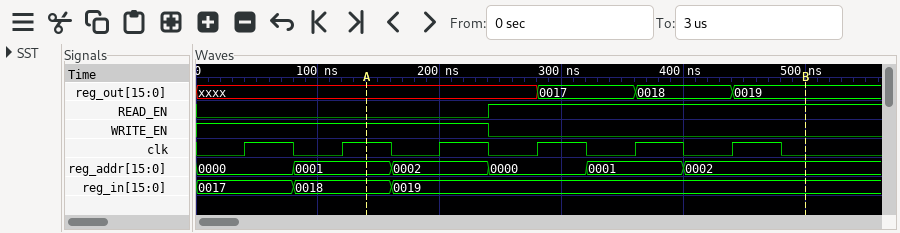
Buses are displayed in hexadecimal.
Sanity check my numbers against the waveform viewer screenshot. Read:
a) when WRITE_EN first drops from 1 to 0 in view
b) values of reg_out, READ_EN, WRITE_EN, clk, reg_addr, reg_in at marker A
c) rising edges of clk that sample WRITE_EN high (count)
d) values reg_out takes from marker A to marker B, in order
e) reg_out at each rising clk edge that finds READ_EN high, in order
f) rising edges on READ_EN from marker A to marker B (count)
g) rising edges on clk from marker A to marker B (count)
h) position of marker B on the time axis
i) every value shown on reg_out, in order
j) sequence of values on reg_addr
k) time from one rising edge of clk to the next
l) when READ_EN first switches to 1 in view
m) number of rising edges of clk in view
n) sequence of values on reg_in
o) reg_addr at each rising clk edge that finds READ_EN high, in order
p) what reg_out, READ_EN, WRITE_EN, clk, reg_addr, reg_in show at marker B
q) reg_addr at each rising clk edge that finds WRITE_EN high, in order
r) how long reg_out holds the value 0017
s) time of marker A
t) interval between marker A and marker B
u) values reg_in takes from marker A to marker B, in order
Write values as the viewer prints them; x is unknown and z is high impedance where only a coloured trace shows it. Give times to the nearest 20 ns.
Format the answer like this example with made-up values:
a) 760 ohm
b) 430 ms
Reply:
a) 240 ns
b) reg_out=xxxx, READ_EN=0, WRITE_EN=1, clk=1, reg_addr=0001, reg_in=0018
c) 3
d) xxxx, 0017, 0018, 0019
e) xxxx, 0017, 0018
f) 1
g) 4
h) 500 ns
i) xxxx, 0017, 0018, 0019
j) 0000, 0001, 0002, 0000, 0001, 0002
k) 80 ns
l) 240 ns
m) 6
n) 0017, 0018, 0019
o) 0000, 0001, 0002
p) reg_out=0019, READ_EN=1, WRITE_EN=0, clk=0, reg_addr=0002, reg_in=0019
q) 0000, 0001, 0002
r) 80 ns
s) 140 ns
t) 360 ns
u) 0018, 0019
